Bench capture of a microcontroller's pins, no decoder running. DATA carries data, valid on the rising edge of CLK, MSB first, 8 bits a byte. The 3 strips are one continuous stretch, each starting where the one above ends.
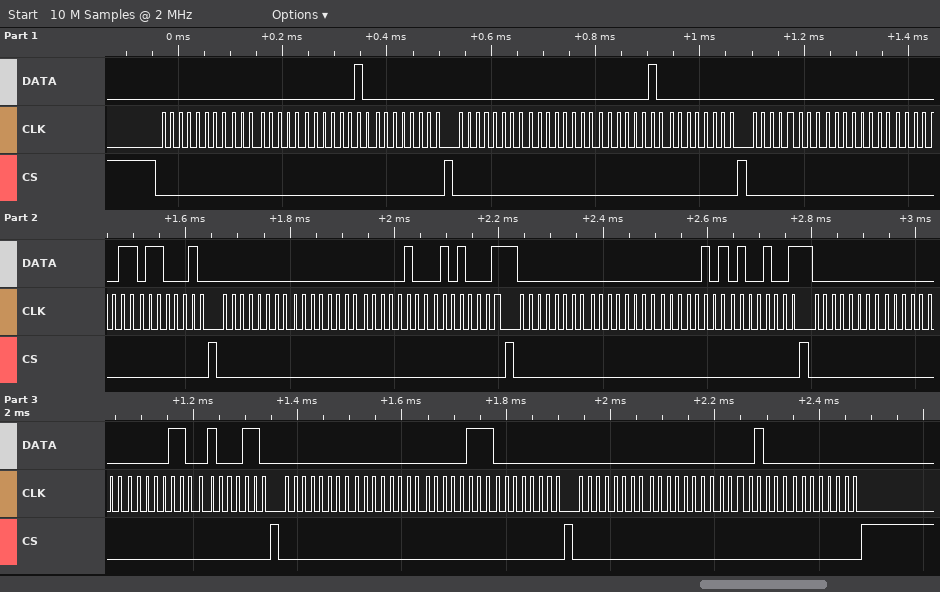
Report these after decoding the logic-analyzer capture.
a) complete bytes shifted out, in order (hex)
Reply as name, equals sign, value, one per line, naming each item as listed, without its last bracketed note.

complete bytes shifted out, in order = 0x00 0x00 0x02 0x00 0x00 0x00 0x02 0x00 0x00 0x00 0x03 0x62 0x00 0x00 0x04 0x51 0x00 0x00 0x05 0x49 0x00 0x00 0x06 0x46 0x00 0x00 0x07 0x00 0x00 0x00 0x08 0x00
